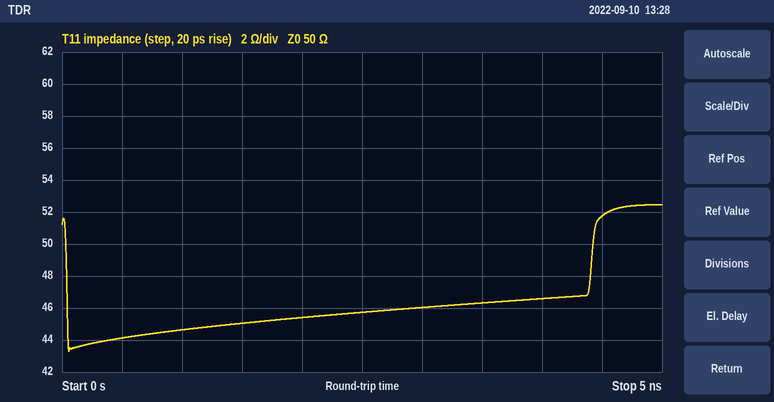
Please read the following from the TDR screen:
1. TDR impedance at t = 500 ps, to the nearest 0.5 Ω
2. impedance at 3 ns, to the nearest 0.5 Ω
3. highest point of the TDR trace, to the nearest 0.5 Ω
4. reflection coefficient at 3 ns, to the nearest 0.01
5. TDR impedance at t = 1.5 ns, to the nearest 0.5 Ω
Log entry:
44.0 Ω
46.0 Ω
52.5 Ω
-0.04
45.0 Ω
